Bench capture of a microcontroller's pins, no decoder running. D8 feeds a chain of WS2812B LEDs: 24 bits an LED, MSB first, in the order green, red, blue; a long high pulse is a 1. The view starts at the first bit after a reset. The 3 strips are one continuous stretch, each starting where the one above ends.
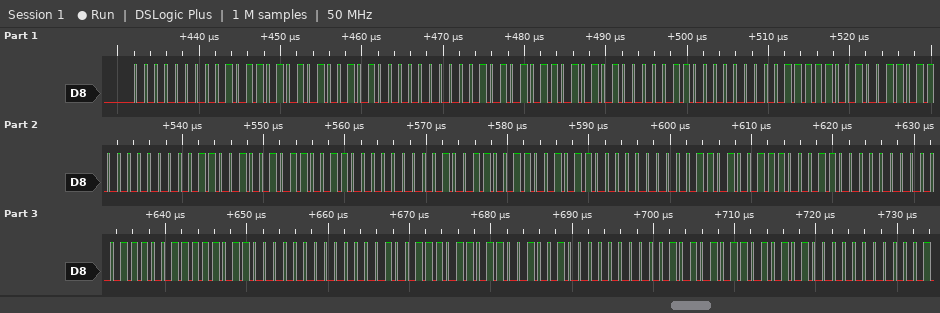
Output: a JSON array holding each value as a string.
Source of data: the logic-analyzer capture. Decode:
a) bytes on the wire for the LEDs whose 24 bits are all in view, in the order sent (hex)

["00 5A A5 00 2A D5 06 00 F9 36 00 C9 66 00 99 96 00 69 C6 00 39 F6 00 09 DB 24 00 AB 54 00"]
